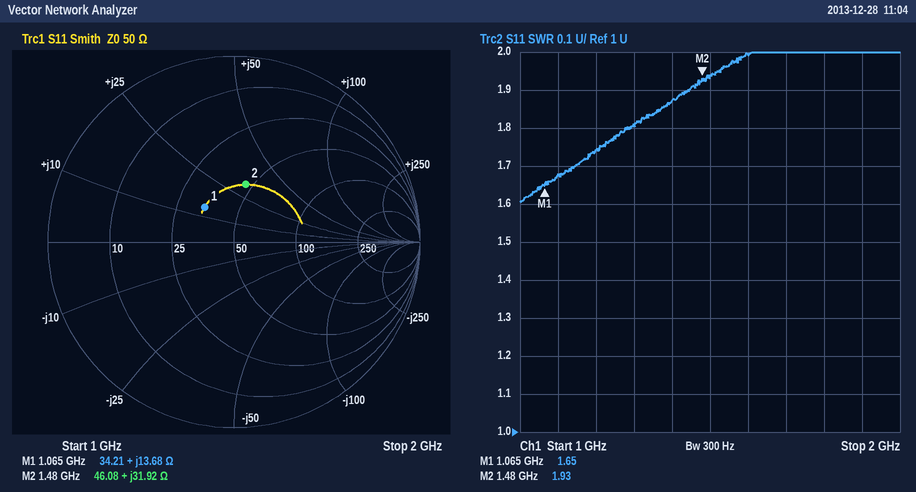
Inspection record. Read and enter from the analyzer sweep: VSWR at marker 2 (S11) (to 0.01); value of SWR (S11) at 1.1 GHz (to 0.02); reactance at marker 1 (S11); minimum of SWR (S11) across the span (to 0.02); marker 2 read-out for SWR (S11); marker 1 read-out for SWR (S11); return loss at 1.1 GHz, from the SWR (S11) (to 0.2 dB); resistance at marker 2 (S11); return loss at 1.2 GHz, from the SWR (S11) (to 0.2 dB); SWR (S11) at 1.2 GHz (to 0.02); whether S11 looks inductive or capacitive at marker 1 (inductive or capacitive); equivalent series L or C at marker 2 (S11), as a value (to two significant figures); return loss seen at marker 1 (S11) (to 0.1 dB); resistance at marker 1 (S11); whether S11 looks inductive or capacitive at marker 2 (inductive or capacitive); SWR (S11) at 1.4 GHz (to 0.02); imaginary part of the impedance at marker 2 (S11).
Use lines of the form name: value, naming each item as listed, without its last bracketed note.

VSWR at marker 2 (S11): 1.93
value of SWR (S11) at 1.1 GHz: 1.68
reactance at marker 1: +13.68 Ω
minimum of SWR (S11) across the span: 1.60
marker 2 read-out for SWR: 1.93
marker 1 read-out for SWR: 1.65
return loss at 1.1 GHz, from the SWR (S11): 12.0 dB
resistance at marker 2: 46.08 Ω
return loss at 1.2 GHz, from the SWR (S11): 11.4 dB
SWR (S11) at 1.2 GHz: 1.74
whether S11 looks inductive or capacitive at marker 1: inductive
equivalent series L or C at marker 2 (S11), as a value: 3.4 nH
return loss seen at marker 1 (S11): 12.2 dB
resistance at marker 1: 34.21 Ω
whether S11 looks inductive or capacitive at marker 2: inductive
SWR (S11) at 1.4 GHz: 1.88
imaginary part of the impedance at marker 2: +31.92 Ω
